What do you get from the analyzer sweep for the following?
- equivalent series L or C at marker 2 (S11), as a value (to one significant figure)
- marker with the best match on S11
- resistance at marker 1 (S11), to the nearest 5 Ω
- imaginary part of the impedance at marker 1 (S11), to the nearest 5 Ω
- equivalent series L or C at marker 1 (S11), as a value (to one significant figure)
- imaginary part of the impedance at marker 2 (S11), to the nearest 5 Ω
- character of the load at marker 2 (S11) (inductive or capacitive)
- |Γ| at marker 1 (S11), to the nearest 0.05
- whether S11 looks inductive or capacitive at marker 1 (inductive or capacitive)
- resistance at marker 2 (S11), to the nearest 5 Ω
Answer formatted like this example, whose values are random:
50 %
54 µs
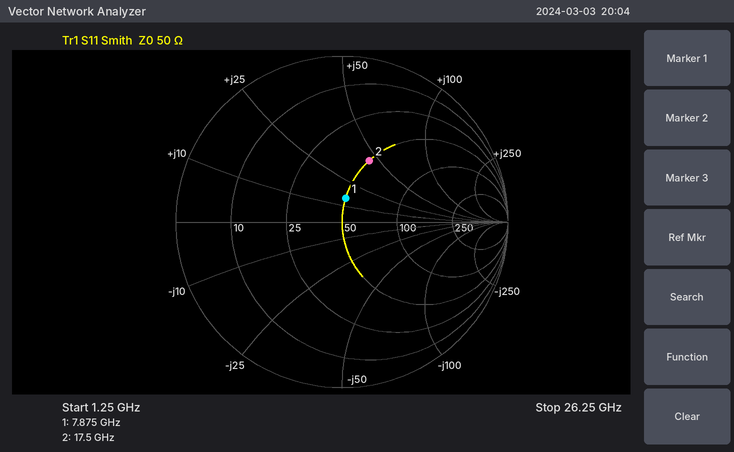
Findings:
400 pH
marker 1
50 Ω
+15 Ω
300 pH
+45 Ω
inductive
0.15
inductive
50 Ω
